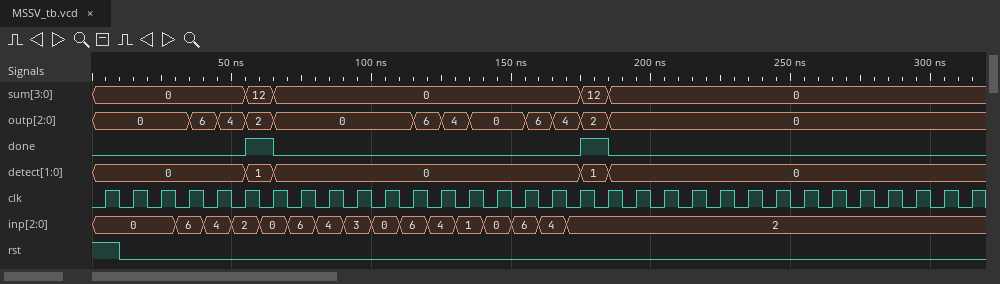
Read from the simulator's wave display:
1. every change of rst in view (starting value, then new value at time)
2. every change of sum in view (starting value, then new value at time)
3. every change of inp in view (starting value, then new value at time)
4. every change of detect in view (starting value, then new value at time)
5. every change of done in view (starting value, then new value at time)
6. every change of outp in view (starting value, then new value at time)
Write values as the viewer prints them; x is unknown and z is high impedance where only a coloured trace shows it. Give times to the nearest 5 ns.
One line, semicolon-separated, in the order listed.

1, 0 at 10 ns; 0, 12 at 55 ns, 0 at 65 ns, 12 at 175 ns, 0 at 185 ns; 0, 6 at 30 ns, 4 at 40 ns, 2 at 50 ns, 0 at 60 ns, 6 at 70 ns, 4 at 80 ns, 3 at 90 ns, 0 at 100 ns, 6 at 110 ns, 4 at 120 ns, 1 at 130 ns, 0 at 140 ns, 6 at 150 ns, 4 at 160 ns, 2 at 170 ns; 0, 1 at 55 ns, 0 at 65 ns, 1 at 175 ns, 0 at 185 ns; 0, 1 at 55 ns, 0 at 65 ns, 1 at 175 ns, 0 at 185 ns; 0, 6 at 35 ns, 4 at 45 ns, 2 at 55 ns, 0 at 65 ns, 6 at 115 ns, 4 at 125 ns, 0 at 135 ns, 6 at 155 ns, 4 at 165 ns, 2 at 175 ns, 0 at 185 ns
